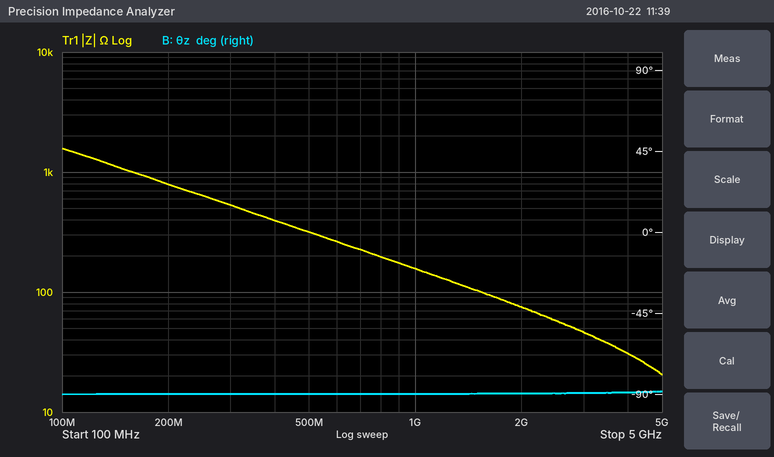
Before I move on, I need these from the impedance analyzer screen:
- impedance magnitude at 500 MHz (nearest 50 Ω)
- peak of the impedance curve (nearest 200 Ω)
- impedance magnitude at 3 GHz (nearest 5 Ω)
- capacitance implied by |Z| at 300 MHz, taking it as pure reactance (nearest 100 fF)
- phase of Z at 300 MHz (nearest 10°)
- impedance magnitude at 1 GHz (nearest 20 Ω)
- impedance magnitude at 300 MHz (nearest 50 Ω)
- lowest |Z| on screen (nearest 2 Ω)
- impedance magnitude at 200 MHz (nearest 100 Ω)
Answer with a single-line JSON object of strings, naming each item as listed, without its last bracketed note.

{"impedance magnitude at 500 MHz": "300 Ω", "peak of the impedance curve": "1.6 kΩ", "impedance magnitude at 3 GHz": "45 Ω", "capacitance implied by |Z| at 300 MHz, taking it as pure reactance": "1.0 pF", "phase of Z at 300 MHz": "-90°", "impedance magnitude at 1 GHz": "160 Ω", "impedance magnitude at 300 MHz": "550 Ω", "lowest |Z| on screen": "20 Ω", "impedance magnitude at 200 MHz": "800 Ω"}
